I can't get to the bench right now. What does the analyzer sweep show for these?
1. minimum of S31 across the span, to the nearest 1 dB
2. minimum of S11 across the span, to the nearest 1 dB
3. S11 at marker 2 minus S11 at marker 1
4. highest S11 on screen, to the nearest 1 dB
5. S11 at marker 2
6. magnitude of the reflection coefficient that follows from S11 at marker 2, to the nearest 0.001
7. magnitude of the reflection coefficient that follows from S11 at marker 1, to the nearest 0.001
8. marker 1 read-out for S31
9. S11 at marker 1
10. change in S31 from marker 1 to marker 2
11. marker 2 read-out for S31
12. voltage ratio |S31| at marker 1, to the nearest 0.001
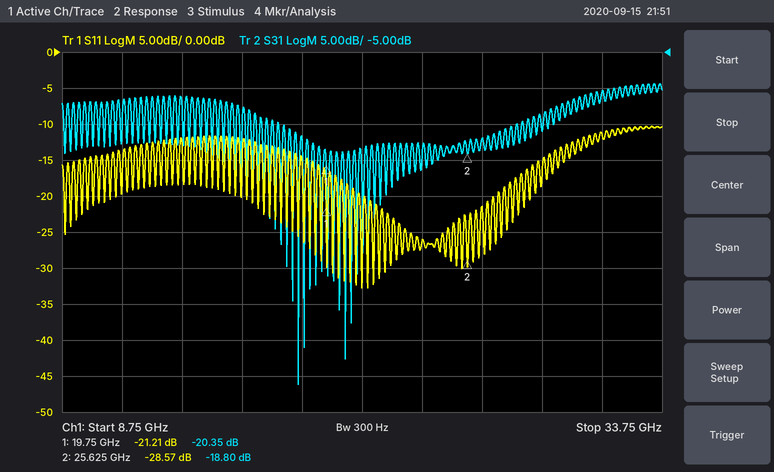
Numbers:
-51 dB
-33 dB
-7.36 dB
-10 dB
-28.57 dB
0.037
0.087
-20.35 dB
-21.21 dB
1.55 dB
-18.80 dB
0.096
